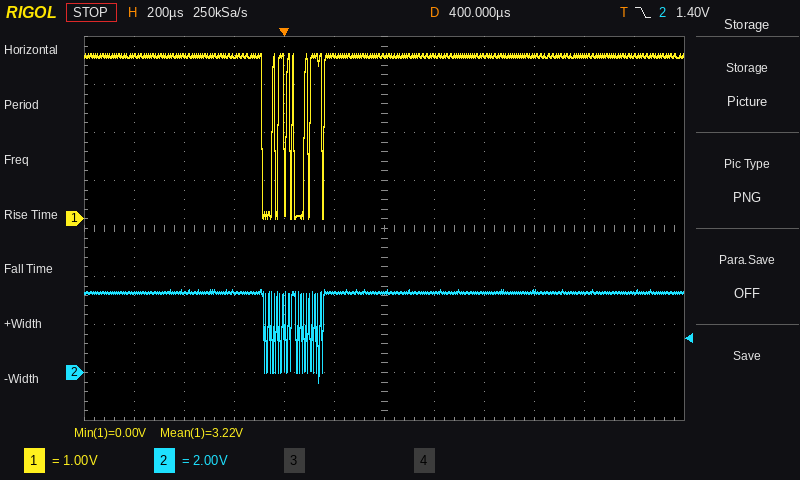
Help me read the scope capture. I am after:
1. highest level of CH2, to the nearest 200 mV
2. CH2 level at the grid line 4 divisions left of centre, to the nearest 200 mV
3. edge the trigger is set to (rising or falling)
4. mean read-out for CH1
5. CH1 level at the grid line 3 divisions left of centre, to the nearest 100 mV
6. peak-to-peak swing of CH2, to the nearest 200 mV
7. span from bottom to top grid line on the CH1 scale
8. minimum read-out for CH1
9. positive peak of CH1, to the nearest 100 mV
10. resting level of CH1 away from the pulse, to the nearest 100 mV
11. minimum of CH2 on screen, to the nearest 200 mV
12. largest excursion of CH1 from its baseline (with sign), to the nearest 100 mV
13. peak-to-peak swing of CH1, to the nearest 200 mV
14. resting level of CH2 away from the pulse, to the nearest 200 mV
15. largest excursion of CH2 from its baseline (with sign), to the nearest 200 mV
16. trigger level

3.4 V
3.4 V
falling
3.22 V
3.4 V
3.8 V
8 V
0.00 V
3.4 V
3.4 V
-400 mV
-3.4 V
3.4 V
3.4 V
-3.8 V
1.40 V
